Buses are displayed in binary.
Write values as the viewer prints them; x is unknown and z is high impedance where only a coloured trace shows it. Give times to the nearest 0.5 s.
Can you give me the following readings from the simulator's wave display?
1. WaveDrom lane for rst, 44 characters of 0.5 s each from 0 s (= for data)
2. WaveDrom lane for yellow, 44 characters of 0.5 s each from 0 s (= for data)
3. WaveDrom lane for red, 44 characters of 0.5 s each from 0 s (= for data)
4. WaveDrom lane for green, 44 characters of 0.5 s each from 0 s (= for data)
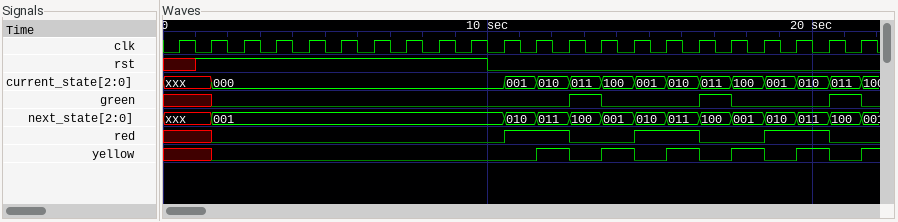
{name: 'rst', wave: 'x.1.................0.......................'}
{name: 'yellow', wave: 'x..0...................1.0.1.0.1.0.1.0.1.0.1'}
{name: 'red', wave: 'x..0.................1...0...1...0...1...0..'}
{name: 'green', wave: 'x..0.....................1.0.....1.0.....1.0'}
